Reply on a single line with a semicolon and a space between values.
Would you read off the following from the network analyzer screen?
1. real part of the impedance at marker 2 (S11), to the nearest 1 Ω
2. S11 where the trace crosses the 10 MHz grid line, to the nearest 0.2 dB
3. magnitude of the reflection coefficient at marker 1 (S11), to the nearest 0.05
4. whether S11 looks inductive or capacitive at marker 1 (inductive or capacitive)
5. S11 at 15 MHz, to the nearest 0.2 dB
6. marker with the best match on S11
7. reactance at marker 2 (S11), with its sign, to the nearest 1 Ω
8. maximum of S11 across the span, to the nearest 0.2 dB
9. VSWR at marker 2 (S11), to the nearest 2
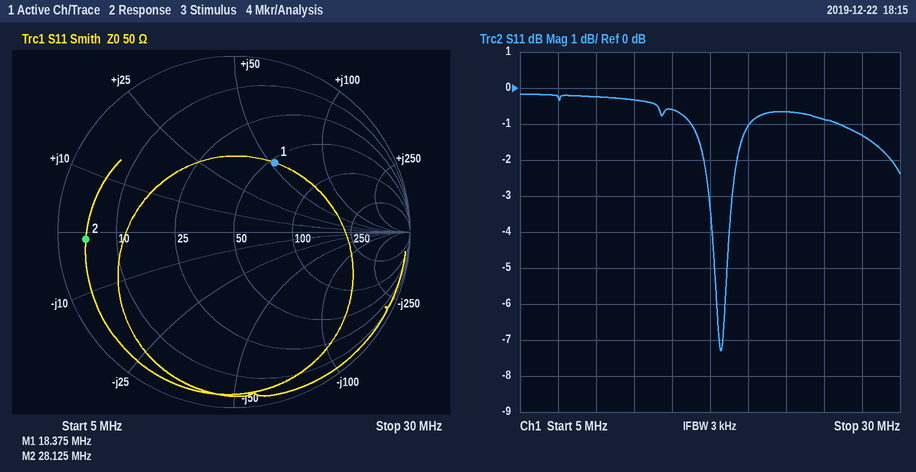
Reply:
4 Ω; -0.2 dB; 0.45; inductive; -0.6 dB; marker 1; -1 Ω; -0.2 dB; 12
